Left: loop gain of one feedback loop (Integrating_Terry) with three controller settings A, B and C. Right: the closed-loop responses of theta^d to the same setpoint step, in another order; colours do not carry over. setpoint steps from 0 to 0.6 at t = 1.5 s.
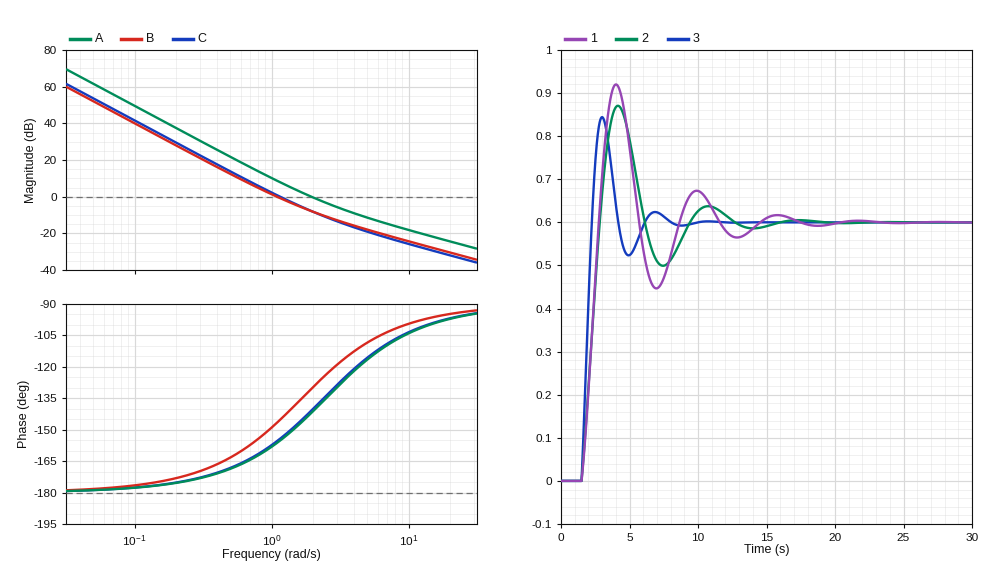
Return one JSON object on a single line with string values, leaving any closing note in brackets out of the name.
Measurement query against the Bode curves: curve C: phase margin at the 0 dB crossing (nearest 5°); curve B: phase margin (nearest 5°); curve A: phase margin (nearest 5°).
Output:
{"curve C: phase margin at the 0 dB crossing": "25°", "curve B: phase margin": "35°", "curve A: phase margin": "40°"}
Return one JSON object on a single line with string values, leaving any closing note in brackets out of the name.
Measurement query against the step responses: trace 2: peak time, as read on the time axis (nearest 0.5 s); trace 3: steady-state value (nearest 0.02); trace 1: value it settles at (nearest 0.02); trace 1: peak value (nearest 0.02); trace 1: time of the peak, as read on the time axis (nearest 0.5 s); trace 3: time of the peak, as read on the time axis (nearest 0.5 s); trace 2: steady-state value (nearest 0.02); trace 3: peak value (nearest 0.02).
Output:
{"trace 2: peak time, as read on the time axis": "4.0 s", "trace 3: steady-state value": "0.60", "trace 1: value it settles at": "0.60", "trace 1: peak value": "0.92", "trace 1: time of the peak, as read on the time axis": "4.0 s", "trace 3: time of the peak, as read on the time axis": "3.0 s", "trace 2: steady-state value": "0.60", "trace 3: peak value": "0.84"}
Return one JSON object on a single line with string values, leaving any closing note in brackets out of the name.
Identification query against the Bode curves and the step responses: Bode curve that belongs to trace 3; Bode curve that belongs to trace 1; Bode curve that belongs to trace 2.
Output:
{"Bode curve that belongs to trace 3": "A", "Bode curve that belongs to trace 1": "C", "Bode curve that belongs to trace 2": "B"}
